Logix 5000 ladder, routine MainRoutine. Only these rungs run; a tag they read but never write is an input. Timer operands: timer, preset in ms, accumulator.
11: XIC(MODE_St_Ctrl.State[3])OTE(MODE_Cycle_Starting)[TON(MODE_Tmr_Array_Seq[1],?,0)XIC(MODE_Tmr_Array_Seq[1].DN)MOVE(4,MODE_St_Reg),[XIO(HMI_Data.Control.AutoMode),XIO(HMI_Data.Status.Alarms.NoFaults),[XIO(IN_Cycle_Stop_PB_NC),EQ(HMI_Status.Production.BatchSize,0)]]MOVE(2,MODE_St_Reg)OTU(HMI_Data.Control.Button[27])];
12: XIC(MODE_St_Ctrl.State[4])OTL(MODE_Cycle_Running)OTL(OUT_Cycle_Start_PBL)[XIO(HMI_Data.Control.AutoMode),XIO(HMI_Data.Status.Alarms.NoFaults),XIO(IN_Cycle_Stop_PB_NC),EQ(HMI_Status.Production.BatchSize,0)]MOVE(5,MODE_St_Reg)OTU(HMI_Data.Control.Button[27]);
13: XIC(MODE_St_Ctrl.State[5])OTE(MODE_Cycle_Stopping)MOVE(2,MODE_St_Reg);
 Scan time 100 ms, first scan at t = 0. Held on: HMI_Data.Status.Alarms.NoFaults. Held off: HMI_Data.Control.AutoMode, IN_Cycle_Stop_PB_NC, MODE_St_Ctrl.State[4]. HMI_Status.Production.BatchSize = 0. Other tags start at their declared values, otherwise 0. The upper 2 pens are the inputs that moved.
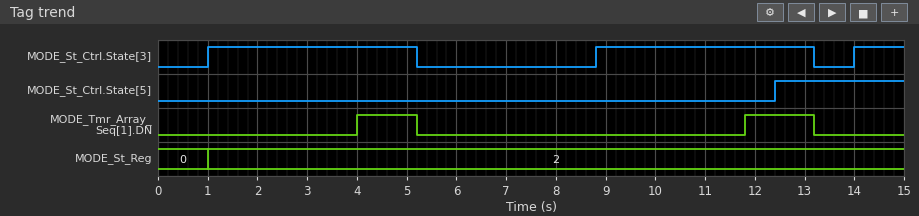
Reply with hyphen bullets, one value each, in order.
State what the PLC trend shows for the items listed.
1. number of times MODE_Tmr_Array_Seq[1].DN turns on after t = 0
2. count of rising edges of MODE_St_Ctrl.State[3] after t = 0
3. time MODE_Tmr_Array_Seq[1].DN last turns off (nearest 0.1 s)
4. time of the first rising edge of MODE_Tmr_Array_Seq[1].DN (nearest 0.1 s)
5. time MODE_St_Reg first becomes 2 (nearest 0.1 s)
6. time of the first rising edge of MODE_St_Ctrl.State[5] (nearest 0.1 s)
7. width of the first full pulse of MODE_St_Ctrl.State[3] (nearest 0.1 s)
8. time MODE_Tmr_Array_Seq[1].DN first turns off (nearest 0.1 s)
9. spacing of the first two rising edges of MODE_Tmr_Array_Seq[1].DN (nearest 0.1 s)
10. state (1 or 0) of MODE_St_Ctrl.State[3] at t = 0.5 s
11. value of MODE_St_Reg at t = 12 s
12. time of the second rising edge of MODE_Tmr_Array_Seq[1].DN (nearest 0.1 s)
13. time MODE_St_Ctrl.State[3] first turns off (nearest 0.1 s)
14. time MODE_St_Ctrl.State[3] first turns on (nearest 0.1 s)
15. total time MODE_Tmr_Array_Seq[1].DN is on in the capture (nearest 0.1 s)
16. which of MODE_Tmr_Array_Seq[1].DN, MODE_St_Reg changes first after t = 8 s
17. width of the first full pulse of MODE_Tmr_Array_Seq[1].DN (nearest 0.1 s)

- 2
- 3
- 13.2 s
- 4.0 s
- 1.0 s
- 12.4 s
- 4.2 s
- 5.2 s
- 7.8 s
- 0
- 2
- 11.8 s
- 5.2 s
- 1.0 s
- 2.6 s
- MODE_Tmr_Array_Seq[1].DN
- 1.2 s
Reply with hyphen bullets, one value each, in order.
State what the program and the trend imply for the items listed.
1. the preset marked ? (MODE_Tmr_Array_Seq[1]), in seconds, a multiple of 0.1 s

- 3.0 s
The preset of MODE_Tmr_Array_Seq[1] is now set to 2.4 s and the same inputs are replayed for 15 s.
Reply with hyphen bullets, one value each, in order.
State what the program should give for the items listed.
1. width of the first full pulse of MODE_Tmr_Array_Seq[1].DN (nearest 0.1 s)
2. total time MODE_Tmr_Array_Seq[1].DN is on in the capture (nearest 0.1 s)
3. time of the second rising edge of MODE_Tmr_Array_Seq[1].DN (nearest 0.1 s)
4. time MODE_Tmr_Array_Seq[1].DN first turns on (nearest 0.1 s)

- 1.8 s
- 3.8 s
- 11.2 s
- 3.4 s
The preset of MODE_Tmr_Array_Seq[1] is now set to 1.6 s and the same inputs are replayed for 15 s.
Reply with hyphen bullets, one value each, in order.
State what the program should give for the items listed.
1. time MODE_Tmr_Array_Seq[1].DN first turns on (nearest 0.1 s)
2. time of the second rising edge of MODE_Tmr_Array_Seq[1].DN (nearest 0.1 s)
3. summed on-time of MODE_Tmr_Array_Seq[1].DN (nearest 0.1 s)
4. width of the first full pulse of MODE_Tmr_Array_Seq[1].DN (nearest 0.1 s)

- 2.6 s
- 10.4 s
- 5.4 s
- 2.6 s
